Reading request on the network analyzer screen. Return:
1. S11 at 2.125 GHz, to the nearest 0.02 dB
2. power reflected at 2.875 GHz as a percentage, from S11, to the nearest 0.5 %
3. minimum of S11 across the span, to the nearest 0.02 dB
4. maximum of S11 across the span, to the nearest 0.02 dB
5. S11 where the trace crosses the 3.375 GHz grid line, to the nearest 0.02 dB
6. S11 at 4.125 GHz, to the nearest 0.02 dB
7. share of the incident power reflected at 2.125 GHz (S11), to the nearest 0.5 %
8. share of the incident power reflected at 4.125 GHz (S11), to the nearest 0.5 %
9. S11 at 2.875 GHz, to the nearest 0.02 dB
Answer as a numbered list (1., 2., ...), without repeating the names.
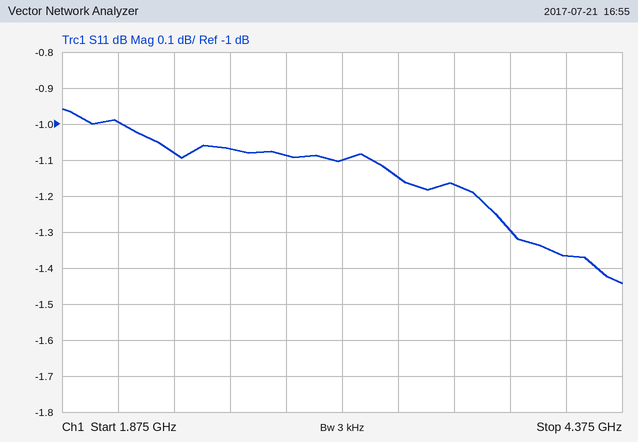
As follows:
1. -1.00 dB
2. 78.0 %
3. -1.44 dB
4. -0.96 dB
5. -1.14 dB
6. -1.36 dB
7. 79.5 %
8. 73.0 %
9. -1.08 dB
